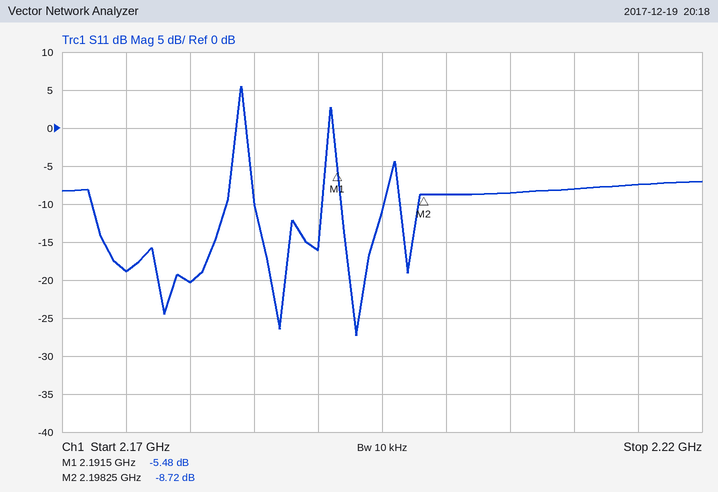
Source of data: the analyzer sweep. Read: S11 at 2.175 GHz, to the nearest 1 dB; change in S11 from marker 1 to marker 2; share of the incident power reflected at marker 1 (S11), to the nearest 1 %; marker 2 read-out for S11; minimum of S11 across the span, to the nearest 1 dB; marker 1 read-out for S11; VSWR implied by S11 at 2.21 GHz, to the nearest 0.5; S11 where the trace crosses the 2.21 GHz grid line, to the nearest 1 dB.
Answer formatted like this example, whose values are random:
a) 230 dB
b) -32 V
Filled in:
a) -19 dB
b) -3.24 dB
c) 28 %
d) -8.72 dB
e) -27 dB
f) -5.48 dB
g) 2.5
h) -8 dB
